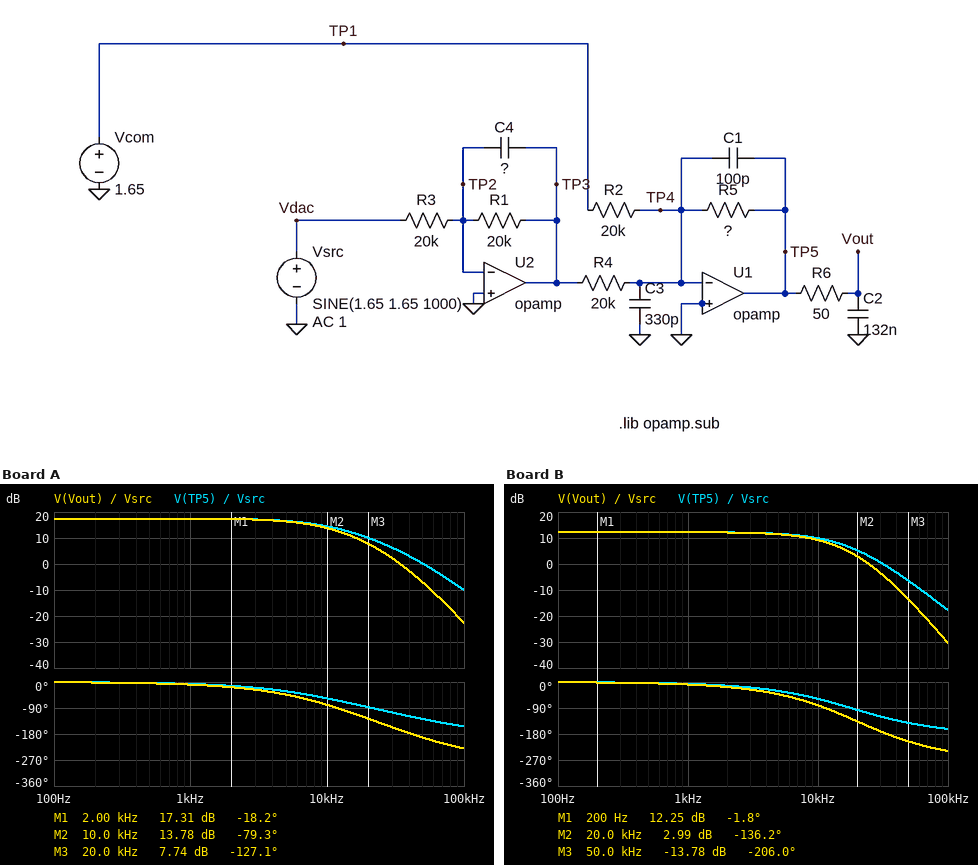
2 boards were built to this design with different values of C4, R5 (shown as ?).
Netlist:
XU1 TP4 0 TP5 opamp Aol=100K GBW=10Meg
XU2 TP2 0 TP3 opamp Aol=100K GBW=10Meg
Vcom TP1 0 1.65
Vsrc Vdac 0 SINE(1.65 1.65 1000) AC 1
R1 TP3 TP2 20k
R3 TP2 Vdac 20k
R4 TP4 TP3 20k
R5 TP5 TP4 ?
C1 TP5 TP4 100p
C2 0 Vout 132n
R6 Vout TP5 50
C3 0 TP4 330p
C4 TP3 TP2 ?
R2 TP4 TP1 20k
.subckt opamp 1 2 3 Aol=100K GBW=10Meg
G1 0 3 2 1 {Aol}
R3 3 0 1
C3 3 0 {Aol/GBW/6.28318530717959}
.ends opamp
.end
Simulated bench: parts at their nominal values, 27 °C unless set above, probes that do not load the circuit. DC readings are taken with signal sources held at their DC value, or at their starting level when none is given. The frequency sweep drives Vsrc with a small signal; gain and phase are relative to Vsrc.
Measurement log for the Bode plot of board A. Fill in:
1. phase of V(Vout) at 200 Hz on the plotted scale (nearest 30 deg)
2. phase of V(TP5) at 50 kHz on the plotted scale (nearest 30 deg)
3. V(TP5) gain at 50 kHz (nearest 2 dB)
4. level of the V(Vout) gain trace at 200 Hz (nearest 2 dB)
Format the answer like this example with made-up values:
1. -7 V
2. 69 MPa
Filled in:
1. 0 deg
2. -120 deg
3. 0 dB
4. 18 dB
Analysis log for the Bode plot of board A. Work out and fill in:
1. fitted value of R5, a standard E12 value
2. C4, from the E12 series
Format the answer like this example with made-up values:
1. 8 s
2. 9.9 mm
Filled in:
1. 150 kΩ
2. 180 pF
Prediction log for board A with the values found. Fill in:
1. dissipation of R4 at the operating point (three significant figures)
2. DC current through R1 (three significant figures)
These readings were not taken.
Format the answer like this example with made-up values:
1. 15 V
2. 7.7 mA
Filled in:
1. 136 µW
2. 82.5 µA
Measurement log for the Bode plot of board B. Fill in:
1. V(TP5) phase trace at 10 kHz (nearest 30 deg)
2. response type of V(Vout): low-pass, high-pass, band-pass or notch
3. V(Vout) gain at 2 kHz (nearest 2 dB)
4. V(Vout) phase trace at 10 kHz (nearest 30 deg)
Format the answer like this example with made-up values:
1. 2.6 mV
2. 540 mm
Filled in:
1. -60 deg
2. low-pass
3. 12 dB
4. -90 deg
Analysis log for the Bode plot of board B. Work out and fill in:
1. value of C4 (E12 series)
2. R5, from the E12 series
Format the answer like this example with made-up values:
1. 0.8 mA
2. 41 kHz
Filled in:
1. 470 pF
2. 82 kΩ
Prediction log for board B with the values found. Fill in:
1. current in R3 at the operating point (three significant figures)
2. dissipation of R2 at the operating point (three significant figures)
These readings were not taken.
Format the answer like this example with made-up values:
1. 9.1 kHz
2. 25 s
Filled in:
1. 82.5 µA
2. 136 µW
